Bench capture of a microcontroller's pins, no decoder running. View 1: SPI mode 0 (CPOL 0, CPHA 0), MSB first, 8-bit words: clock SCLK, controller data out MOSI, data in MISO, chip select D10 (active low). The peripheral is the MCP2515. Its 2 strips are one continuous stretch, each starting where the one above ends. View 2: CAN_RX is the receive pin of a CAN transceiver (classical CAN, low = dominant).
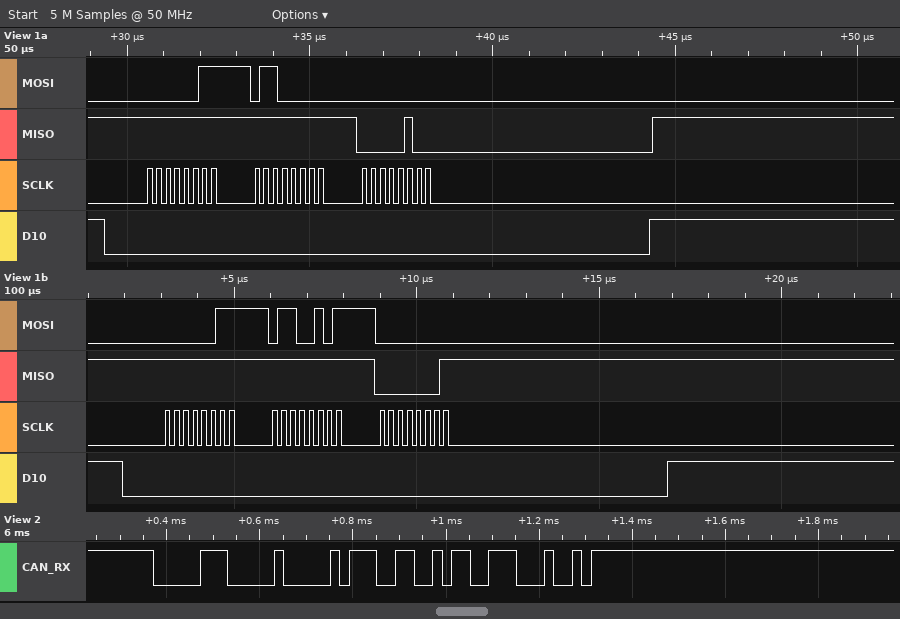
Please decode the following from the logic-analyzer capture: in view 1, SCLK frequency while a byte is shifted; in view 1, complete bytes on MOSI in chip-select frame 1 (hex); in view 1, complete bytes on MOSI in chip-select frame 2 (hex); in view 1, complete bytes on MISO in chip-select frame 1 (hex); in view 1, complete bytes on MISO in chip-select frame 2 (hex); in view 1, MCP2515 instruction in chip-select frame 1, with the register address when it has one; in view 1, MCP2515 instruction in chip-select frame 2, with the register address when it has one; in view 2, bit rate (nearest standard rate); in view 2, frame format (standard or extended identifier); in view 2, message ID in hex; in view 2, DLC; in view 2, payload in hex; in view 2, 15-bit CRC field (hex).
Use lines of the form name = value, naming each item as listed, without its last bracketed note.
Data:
in view 1, SCLK frequency while a byte is shifted = 4 MHz
in view 1, complete bytes on MOSI in chip-select frame 1 = 0x03 0x60 0x00
in view 1, complete bytes on MOSI in chip-select frame 2 = 0x03 0x65 0x00
in view 1, complete bytes on MISO in chip-select frame 1 = 0xFF 0xFF 0x04
in view 1, complete bytes on MISO in chip-select frame 2 = 0xFF 0xFF 0x01
in view 1, MCP2515 instruction in chip-select frame 1, with the register address when it has one = READ 0x60
in view 1, MCP2515 instruction in chip-select frame 2, with the register address when it has one = READ 0x65
in view 2, bit rate = 50 kbit/s
in view 2, frame format = standard
in view 2, message ID in hex = 0x060
in view 2, DLC = 1
in view 2, payload in hex = CC
in view 2, 15-bit CRC field = 0x59C4
